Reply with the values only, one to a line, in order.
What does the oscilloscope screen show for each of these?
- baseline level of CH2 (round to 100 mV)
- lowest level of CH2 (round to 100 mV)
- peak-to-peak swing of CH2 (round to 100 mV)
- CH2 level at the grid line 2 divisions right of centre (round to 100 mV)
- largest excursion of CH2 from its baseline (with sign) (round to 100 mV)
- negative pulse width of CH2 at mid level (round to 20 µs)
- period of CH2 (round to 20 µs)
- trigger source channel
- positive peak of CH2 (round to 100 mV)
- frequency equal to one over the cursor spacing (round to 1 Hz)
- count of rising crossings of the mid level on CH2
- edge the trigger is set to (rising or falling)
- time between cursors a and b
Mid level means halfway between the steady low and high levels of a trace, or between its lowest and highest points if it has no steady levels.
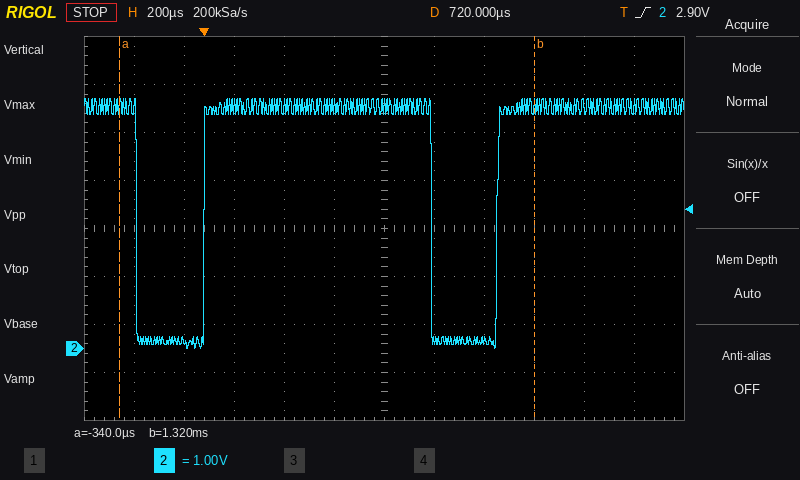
5.0 V
0.0 V
5.2 V
200 mV
-5.0 V
260 µs
1.18 ms
CH2
5.2 V
602 Hz
2
rising
1.66 ms
